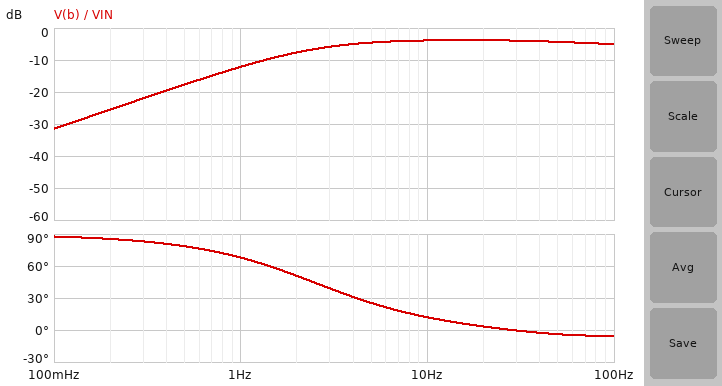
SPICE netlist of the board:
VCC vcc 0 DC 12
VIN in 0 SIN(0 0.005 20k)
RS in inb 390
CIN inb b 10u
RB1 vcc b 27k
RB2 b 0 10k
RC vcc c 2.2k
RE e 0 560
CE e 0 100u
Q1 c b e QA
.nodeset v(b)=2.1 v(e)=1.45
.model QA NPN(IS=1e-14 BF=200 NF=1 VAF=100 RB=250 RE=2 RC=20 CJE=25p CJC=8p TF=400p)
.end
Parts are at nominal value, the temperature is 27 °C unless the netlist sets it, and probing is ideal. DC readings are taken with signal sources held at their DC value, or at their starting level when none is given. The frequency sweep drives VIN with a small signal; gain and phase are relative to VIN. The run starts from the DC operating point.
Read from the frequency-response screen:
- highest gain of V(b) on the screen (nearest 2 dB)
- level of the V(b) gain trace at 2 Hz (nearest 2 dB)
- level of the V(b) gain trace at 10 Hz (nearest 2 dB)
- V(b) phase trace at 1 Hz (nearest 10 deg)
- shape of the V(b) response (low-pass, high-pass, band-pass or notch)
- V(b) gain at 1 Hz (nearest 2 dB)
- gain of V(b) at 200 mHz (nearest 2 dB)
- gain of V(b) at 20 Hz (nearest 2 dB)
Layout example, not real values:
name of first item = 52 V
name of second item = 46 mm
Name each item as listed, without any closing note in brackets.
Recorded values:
highest gain of V(b) on the screen = -4 dB
level of the V(b) gain trace at 2 Hz = -8 dB
level of the V(b) gain trace at 10 Hz = -4 dB
V(b) phase trace at 1 Hz = 70 deg
shape of the V(b) response = high-pass
V(b) gain at 1 Hz = -12 dB
gain of V(b) at 200 mHz = -26 dB
gain of V(b) at 20 Hz = -4 dB
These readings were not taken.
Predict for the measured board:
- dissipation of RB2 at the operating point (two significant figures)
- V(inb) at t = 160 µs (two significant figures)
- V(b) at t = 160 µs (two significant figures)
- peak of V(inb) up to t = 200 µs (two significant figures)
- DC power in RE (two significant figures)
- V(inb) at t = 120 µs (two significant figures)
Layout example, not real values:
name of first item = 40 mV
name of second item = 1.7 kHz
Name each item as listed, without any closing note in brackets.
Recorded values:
dissipation of RB2 at the operating point = 950 µW
V(inb) at t = 160 µs = 1.9 mV
V(b) at t = 160 µs = 3.1 V
peak of V(inb) up to t = 200 µs = 2.1 mV
DC power in RE = 10 mW
V(inb) at t = 120 µs = 1.2 mV
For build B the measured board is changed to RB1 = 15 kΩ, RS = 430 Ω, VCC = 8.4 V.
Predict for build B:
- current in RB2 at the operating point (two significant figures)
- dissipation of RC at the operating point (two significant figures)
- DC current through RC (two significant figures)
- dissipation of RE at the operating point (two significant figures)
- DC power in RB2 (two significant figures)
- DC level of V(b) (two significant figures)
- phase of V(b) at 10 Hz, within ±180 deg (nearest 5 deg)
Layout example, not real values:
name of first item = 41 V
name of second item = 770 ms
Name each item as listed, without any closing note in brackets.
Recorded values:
current in RB2 at the operating point = 250 µA
dissipation of RC at the operating point = 19 mW
DC current through RC = 3.0 mA
dissipation of RE at the operating point = 5.4 mW
DC power in RB2 = 610 µW
DC level of V(b) = 2.5 V
phase of V(b) at 10 Hz, within ±180 deg = 45 deg
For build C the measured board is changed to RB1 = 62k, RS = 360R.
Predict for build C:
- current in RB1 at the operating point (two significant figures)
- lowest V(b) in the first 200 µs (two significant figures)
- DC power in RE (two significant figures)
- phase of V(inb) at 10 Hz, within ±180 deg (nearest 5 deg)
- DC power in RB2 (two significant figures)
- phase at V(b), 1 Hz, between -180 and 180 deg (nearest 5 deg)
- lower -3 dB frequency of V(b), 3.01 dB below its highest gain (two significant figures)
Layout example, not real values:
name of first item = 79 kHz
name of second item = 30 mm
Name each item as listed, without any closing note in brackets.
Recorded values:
current in RB1 at the operating point = 170 µA
lowest V(b) in the first 200 µs = 1.6 V
DC power in RE = 1.5 mW
phase of V(inb) at 10 Hz, within ±180 deg = 0 deg
DC power in RB2 = 260 µW
phase at V(b), 1 Hz, between -180 and 180 deg = 60 deg
lower -3 dB frequency of V(b), 3.01 dB below its highest gain = 1.8 Hz
